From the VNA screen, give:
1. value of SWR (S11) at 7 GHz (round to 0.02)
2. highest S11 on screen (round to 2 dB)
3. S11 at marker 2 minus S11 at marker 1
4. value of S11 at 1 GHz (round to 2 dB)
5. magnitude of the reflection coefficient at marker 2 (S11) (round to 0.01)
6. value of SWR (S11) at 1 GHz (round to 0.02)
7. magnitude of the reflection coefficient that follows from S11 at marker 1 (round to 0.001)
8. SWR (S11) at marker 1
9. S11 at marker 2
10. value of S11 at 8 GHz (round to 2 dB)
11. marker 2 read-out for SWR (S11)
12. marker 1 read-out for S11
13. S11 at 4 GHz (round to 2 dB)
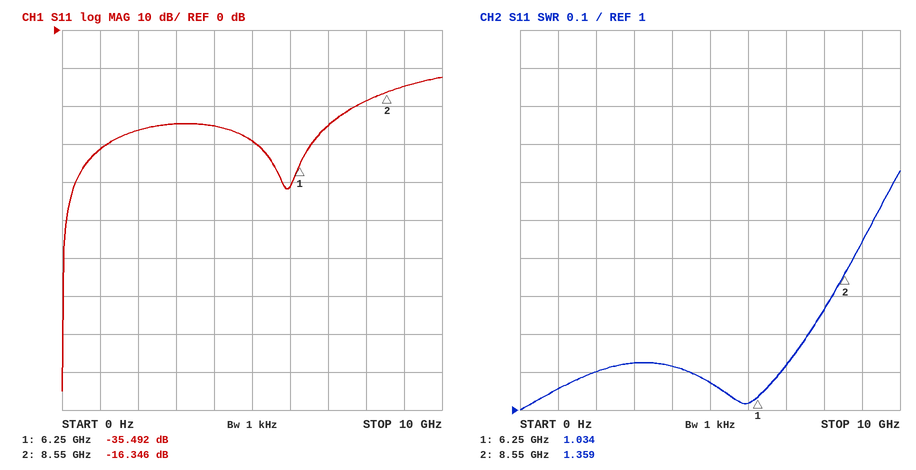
1.12
-12 dB
19.146 dB
-32 dB
0.15
1.06
0.017
1.034
-16.346 dB
-18 dB
1.359
-35.492 dB
-26 dB
